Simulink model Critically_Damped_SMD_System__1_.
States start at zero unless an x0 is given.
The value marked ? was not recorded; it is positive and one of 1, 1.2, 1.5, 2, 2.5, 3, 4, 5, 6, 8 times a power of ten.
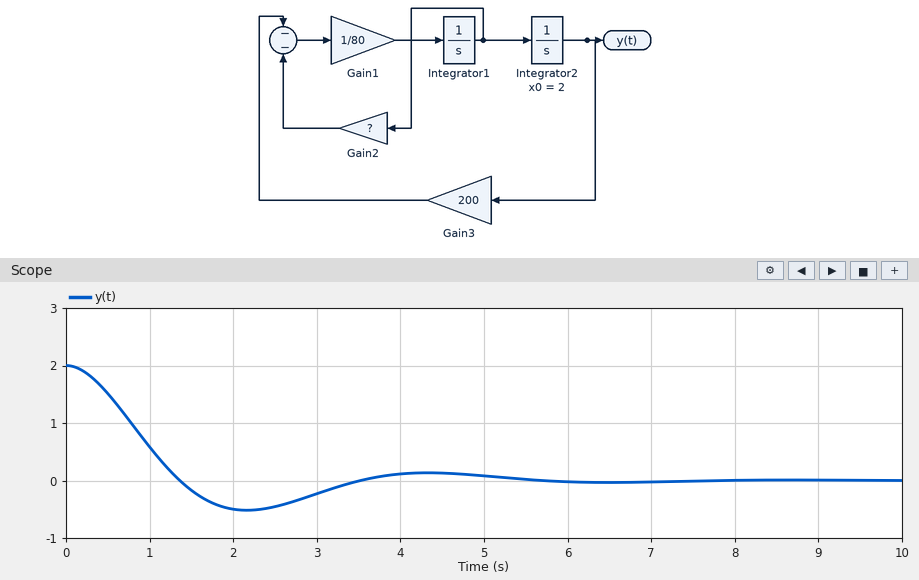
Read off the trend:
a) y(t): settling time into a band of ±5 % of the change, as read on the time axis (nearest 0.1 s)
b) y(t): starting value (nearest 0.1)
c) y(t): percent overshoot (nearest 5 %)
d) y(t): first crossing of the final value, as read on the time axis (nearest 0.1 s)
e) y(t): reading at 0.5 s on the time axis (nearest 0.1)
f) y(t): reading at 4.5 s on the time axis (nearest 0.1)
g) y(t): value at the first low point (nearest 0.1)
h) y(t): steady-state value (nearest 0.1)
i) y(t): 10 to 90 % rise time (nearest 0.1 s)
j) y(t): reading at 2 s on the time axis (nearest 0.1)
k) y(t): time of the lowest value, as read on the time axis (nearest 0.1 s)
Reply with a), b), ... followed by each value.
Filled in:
a) 4.8 s
b) 2.0
c) 25 %
d) 1.4 s
e) 1.5
f) 0.1
g) -0.5
h) 0.0
i) 0.9 s
j) -0.5
k) 2.2 s
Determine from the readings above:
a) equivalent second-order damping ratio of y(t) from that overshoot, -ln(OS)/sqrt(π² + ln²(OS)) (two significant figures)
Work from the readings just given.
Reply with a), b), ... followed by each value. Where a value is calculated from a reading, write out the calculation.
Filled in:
a) ln(0.25) = -1.386; 1.386 / sqrt(9.870 + 1.922) = 0.40
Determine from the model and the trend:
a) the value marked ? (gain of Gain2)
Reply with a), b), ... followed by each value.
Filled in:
a) 100
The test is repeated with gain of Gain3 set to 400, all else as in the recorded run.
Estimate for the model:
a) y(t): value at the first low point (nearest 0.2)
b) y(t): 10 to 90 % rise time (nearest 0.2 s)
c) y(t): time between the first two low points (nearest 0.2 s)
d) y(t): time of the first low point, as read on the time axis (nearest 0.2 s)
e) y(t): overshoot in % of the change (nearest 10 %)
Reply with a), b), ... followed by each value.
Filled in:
a) -0.8
b) 0.6 s
c) 3.0 s
d) 1.4 s
e) 40 %
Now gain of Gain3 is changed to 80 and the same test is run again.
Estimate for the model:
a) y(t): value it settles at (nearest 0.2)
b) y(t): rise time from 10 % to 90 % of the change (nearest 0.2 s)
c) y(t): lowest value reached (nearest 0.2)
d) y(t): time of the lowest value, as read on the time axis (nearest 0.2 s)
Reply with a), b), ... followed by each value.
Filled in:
a) 0.0
b) 2.0 s
c) -0.2
d) 4.0 s
